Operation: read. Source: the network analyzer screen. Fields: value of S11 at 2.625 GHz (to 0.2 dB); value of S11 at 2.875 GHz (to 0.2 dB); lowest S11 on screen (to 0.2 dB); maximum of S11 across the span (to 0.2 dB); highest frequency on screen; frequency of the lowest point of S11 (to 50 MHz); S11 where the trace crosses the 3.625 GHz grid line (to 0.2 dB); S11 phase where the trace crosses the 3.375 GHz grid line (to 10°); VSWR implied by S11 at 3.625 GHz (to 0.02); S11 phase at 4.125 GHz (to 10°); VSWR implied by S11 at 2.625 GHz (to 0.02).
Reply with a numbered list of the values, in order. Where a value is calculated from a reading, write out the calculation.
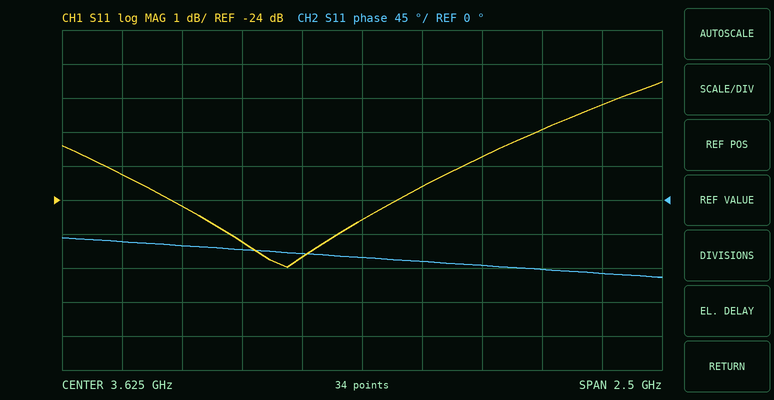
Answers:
1. -23.2 dB
2. -24.2 dB
3. -26.0 dB
4. -20.6 dB
5. 4.875 GHz
6. 3.30 GHz
7. -24.6 dB
8. -70°
9. |Γ| = 10^(-24.6/20) = 0.0589; VSWR = (1 + 0.0589)/(1 − 0.0589) ≈ 1.13, so 1.12 to the nearest 0.02
10. -90°
11. |Γ| = 10^(-23.2/20) = 0.0692; VSWR = (1 + 0.0692)/(1 − 0.0692) ≈ 1.15, so 1.14 to the nearest 0.02
